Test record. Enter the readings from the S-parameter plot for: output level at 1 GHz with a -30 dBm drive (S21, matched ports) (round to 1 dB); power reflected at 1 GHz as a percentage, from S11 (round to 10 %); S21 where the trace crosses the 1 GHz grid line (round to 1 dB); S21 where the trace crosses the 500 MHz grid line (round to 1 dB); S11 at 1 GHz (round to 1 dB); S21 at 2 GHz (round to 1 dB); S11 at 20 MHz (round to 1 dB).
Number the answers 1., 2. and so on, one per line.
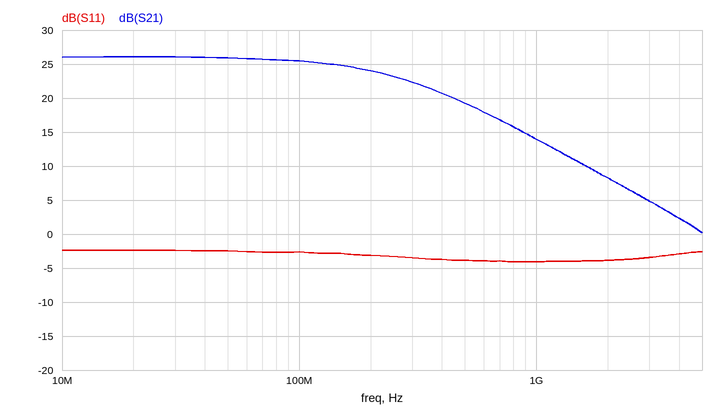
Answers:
1. -16 dBm
2. 40 %
3. 14 dB
4. 19 dB
5. -4 dB
6. 8 dB
7. -2 dB
